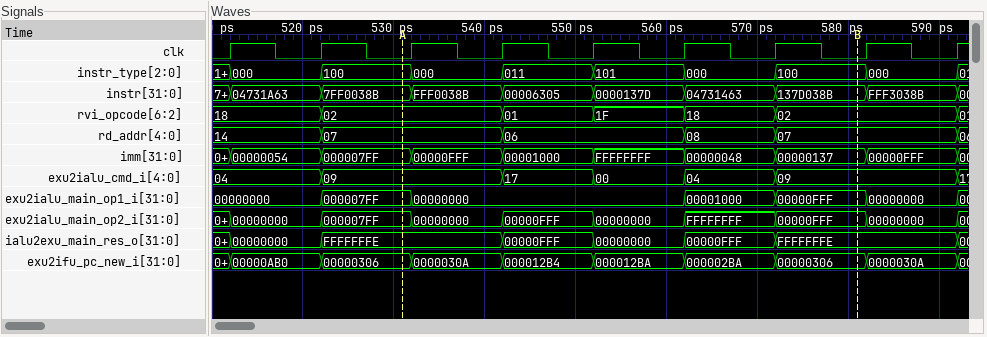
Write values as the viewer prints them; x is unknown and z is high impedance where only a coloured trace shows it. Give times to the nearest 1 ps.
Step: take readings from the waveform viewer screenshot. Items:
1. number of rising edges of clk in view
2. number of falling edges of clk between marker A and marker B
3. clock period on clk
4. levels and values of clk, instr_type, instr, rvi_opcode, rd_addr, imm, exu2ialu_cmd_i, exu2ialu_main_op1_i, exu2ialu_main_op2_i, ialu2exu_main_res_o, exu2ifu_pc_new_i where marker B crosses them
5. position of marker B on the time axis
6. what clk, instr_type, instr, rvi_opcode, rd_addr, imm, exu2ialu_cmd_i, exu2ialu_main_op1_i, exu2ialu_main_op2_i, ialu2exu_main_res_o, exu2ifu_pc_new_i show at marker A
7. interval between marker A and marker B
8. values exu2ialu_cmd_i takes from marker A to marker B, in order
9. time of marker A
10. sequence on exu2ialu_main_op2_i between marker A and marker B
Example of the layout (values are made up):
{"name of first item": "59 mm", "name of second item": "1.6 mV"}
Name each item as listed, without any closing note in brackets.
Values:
{"number of rising edges of clk in view": "9", "number of falling edges of clk between marker A and marker B": "5", "clock period on clk": "10 ps", "levels and values of clk, instr_type, instr, rvi_opcode, rd_addr, imm, exu2ialu_cmd_i, exu2ialu_main_op1_i, exu2ialu_main_op2_i, ialu2exu_main_res_o, exu2ifu_pc_new_i where marker B crosses them": "clk=0, instr_type=100, instr=137D038B, rvi_opcode=02, rd_addr=07, imm=00000137, exu2ialu_cmd_i=09, exu2ialu_main_op1_i=00000FFF, exu2ialu_main_op2_i=00000FFF, ialu2exu_main_res_o=FFFFFFFE, exu2ifu_pc_new_i=00000306", "position of marker B on the time axis": "581 ps", "what clk, instr_type, instr, rvi_opcode, rd_addr, imm, exu2ialu_cmd_i, exu2ialu_main_op1_i, exu2ialu_main_op2_i, ialu2exu_main_res_o, exu2ifu_pc_new_i show at marker A": "clk=0, instr_type=100, instr=7FF0038B, rvi_opcode=02, rd_addr=07, imm=000007FF, exu2ialu_cmd_i=09, exu2ialu_main_op1_i=000007FF, exu2ialu_main_op2_i=000007FF, ialu2exu_main_res_o=FFFFFFFE, exu2ifu_pc_new_i=00000306", "interval between marker A and marker B": "50 ps", "values exu2ialu_cmd_i takes from marker A to marker B, in order": "09, 17, 00, 04, 09", "time of marker A": "531 ps", "sequence on exu2ialu_main_op2_i between marker A and marker B": "000007FF, 00000000, 00000FFF, 00000000, FFFFFFFF, 00000FFF"}
